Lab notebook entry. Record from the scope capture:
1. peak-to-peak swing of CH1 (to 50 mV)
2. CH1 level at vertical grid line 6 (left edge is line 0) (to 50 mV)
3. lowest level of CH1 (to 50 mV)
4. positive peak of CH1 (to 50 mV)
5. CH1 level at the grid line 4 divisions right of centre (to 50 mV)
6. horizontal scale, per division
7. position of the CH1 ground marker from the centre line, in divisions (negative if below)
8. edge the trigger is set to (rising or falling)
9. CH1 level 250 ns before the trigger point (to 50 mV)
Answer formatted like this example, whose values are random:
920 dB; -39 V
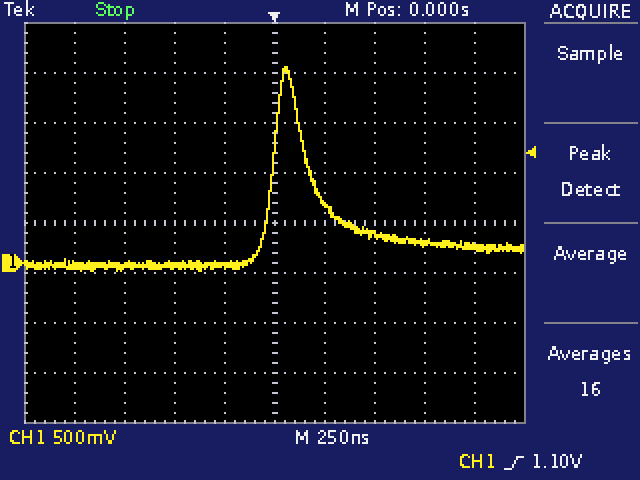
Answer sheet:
2.05 V; 600 mV; -100 mV; 1.95 V; 150 mV; 250 ns; -0.8 div; rising; -50 mV
